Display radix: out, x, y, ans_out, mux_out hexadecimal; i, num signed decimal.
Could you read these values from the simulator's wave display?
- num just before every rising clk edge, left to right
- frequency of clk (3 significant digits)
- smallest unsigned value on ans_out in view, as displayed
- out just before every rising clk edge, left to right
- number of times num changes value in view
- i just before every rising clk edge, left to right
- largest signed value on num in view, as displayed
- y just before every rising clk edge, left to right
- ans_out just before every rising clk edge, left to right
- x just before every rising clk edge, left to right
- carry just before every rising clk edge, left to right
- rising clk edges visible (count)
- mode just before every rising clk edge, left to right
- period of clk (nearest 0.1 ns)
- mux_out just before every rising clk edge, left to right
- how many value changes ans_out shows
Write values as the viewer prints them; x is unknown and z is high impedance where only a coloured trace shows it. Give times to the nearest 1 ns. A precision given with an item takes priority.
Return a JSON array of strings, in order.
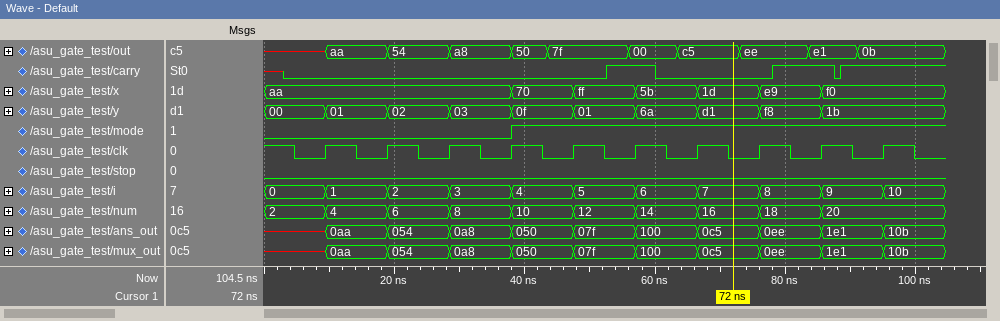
["2, 4, 6, 8, 10, 12, 14, 16, 18, 20", "105 MHz", "050", "x, aa, 54, a8, 7f, 00, c5, ee, e1, 0b", "9", "0, 1, 2, 3, 4, 5, 6, 7, 8, 9", "20", "00, 01, 02, 03, 0f, 01, 6a, d1, f8, 1b", "x, 0aa, 054, 0a8, 050, 07f, 100, 0c5, 0ee, 1e1", "aa, aa, aa, aa, 70, ff, 5b, 1d, e9, f0", "0 0 0 0 0 1 0 0 1 1", "10", "0 0 0 0 1 1 1 1 1 1", "9.5 ns", "x, 0aa, 054, 0a8, 050, 07f, 100, 0c5, 0ee, 1e1", "10"]
